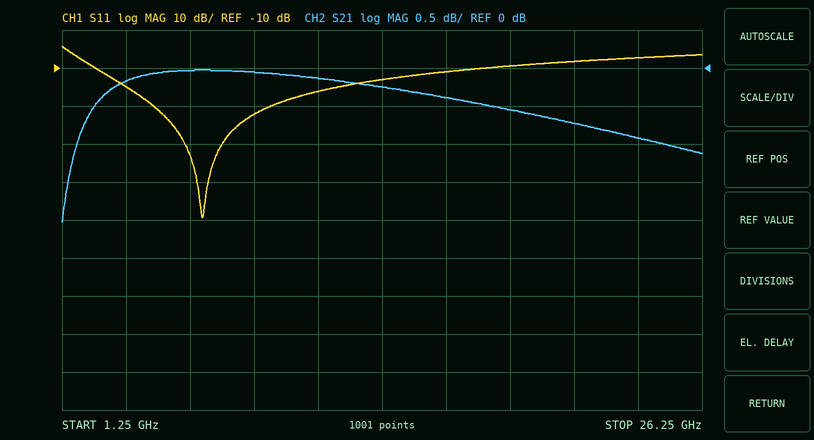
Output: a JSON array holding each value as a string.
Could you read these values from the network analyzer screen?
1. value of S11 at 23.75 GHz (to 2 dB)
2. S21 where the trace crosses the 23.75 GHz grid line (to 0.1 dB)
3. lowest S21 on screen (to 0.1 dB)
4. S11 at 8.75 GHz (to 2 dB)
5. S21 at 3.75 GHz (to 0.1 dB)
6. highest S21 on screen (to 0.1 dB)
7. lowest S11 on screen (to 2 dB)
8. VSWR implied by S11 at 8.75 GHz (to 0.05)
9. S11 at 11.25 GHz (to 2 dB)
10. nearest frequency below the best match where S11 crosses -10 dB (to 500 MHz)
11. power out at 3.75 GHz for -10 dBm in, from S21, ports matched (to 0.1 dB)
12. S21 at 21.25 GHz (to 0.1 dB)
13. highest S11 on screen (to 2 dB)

["-8 dB", "-0.9 dB", "-2.0 dB", "-22 dB", "-0.2 dB", "0.0 dB", "-50 dB", "1.15", "-16 dB", "2.5 GHz", "-10.2 dBm", "-0.7 dB", "-4 dB"]
